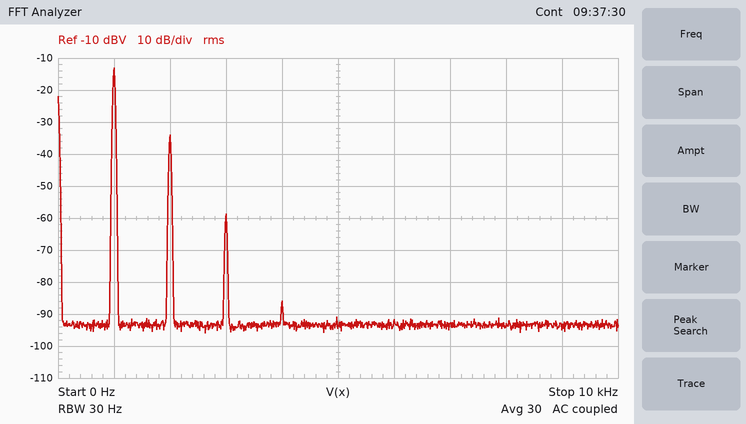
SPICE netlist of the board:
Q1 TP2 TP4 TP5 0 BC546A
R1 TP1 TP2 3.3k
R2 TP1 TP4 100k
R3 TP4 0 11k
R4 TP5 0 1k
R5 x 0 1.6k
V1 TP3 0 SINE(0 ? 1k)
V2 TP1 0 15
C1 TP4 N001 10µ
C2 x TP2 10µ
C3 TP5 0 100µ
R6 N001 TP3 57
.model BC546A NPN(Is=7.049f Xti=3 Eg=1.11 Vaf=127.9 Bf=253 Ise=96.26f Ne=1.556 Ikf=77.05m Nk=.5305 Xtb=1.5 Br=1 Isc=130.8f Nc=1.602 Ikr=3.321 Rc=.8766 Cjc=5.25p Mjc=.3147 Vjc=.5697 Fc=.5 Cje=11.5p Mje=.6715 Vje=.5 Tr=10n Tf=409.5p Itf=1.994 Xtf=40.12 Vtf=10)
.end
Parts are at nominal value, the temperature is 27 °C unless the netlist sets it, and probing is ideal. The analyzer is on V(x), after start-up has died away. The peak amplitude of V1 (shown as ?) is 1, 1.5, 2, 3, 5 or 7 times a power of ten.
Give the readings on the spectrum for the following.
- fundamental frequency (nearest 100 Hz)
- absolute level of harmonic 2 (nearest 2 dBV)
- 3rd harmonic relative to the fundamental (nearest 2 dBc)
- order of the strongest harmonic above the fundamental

1.0 kHz
-34 dBV
-46 dBc
2
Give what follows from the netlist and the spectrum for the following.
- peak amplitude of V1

10 mV
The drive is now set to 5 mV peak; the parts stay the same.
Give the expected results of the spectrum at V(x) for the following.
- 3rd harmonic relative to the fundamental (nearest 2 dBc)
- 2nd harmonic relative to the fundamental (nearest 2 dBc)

-58 dBc
-26 dBc
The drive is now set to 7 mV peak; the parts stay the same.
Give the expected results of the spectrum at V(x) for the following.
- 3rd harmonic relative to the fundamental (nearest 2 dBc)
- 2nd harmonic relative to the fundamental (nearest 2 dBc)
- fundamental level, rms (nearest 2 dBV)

-52 dBc
-24 dBc
-16 dBV
